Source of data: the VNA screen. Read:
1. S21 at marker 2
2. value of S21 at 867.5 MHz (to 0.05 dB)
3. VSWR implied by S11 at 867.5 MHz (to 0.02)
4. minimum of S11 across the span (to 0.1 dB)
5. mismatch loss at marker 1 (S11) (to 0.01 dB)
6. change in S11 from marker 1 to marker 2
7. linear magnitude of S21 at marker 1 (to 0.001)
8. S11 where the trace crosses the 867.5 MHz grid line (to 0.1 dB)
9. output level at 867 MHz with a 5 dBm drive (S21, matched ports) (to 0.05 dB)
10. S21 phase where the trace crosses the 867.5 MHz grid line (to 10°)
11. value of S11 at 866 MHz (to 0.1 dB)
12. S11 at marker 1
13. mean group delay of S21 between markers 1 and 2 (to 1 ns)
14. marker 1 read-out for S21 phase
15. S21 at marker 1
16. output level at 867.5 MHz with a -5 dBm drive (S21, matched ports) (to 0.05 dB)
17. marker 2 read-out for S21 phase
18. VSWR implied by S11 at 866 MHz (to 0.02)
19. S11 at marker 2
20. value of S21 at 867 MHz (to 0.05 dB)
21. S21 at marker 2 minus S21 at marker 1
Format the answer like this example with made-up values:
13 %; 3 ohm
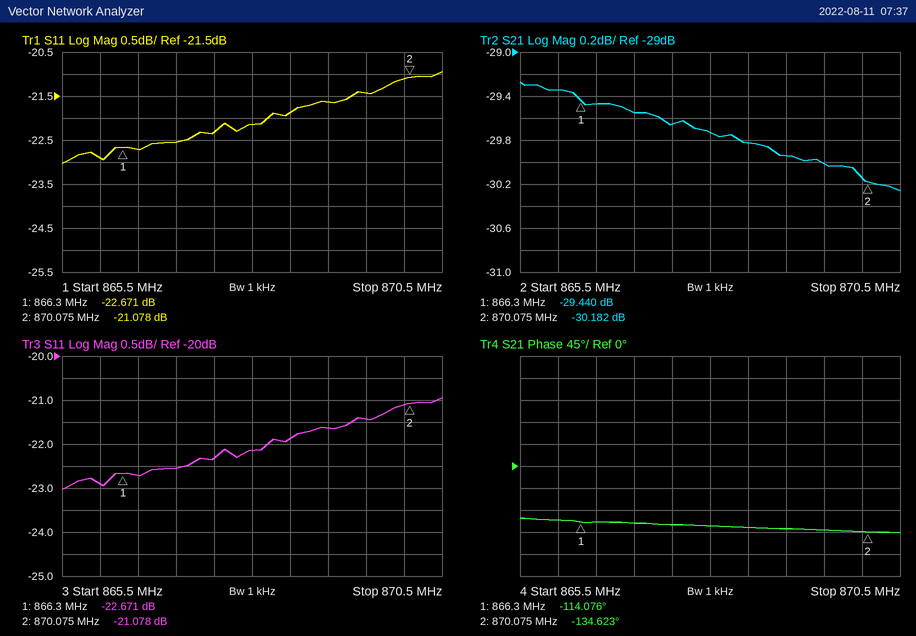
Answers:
-30.182 dB; -29.65 dB; 1.16; -23.0 dB; 0.02 dB; 1.593 dB; 0.034; -22.3 dB; -24.55 dBm; -120°; -22.9 dB; -22.671 dB; 15 ns; -114.076°; -29.440 dB; -34.65 dBm; -134.623°; 1.16; -21.078 dB; -29.55 dB; -0.742 dB
